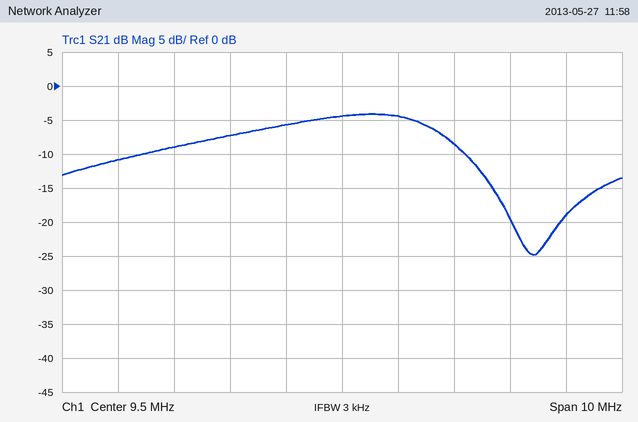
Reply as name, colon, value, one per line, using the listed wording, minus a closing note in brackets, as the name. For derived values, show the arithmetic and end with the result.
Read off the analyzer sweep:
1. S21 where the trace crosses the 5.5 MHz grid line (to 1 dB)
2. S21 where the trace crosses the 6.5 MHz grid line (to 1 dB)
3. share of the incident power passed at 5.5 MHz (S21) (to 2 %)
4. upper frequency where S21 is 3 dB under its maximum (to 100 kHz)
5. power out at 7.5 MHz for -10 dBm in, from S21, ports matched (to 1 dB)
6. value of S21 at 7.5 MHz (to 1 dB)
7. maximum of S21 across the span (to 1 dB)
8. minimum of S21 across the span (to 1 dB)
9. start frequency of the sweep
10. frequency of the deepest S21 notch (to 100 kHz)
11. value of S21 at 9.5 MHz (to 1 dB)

S21 where the trace crosses the 5.5 MHz grid line: -11 dB
S21 where the trace crosses the 6.5 MHz grid line: -9 dB
share of the incident power passed at 5.5 MHz (S21): 10^(-11/10) ≈ 8 %
upper frequency where S21 is 3 dB under its maximum: 11.3 MHz
power out at 7.5 MHz for -10 dBm in, from S21, ports matched: -10 dBm + (-7 dB) = -17 dBm
value of S21 at 7.5 MHz: -7 dB
maximum of S21 across the span: -4 dB
minimum of S21 across the span: -25 dB
start frequency of the sweep: 4.5 MHz
frequency of the deepest S21 notch: 12.9 MHz
value of S21 at 9.5 MHz: -4 dB
